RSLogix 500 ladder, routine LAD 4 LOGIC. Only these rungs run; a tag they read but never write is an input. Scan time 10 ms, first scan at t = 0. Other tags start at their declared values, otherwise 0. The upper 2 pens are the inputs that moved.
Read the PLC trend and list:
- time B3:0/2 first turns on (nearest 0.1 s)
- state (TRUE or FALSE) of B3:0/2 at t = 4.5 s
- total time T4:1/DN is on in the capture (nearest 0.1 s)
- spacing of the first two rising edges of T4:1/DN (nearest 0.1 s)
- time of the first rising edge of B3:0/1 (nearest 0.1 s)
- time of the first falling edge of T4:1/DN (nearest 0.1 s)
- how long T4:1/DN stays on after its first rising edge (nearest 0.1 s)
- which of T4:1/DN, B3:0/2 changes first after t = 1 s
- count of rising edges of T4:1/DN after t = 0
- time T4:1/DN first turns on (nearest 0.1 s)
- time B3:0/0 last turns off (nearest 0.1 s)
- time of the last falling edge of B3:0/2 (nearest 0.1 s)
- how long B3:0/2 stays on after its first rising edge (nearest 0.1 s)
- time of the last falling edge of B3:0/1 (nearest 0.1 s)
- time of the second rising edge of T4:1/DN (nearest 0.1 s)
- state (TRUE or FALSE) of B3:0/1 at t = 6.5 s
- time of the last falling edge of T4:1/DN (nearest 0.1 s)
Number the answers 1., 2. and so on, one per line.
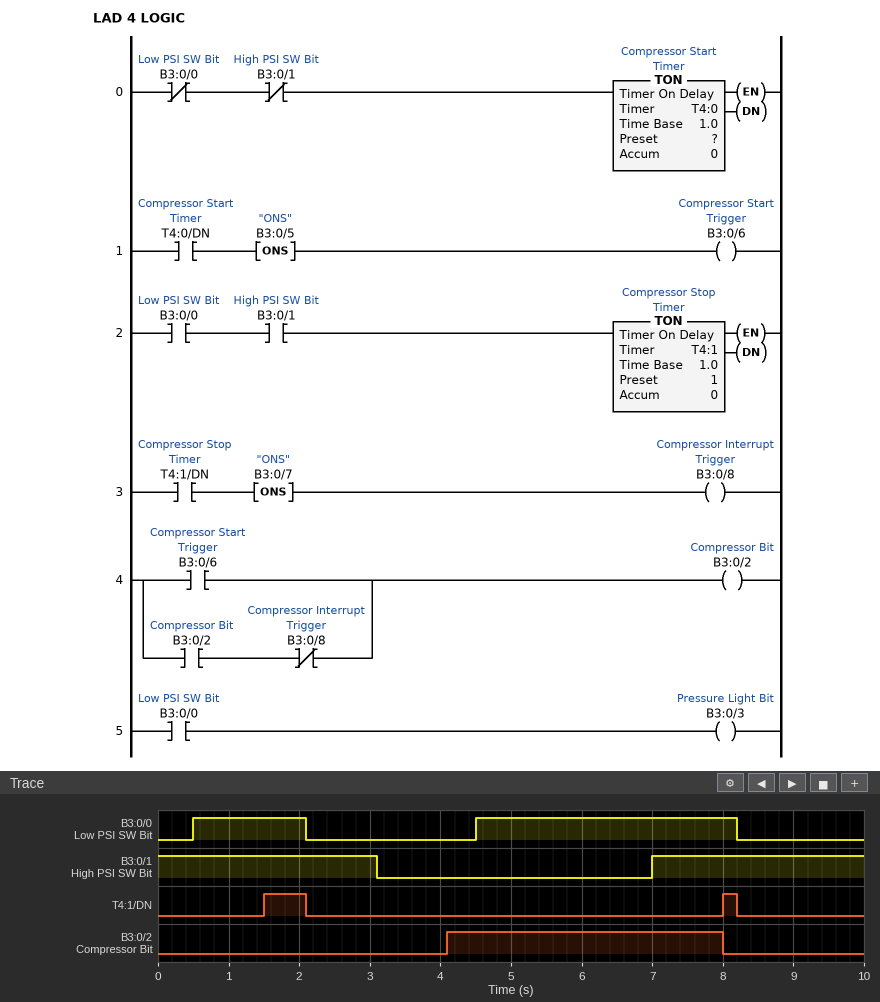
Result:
1. 4.1 s
2. TRUE
3. 0.8 s
4. 6.5 s
5. 7.0 s
6. 2.1 s
7. 0.6 s
8. T4:1/DN
9. 2
10. 1.5 s
11. 8.2 s
12. 8.0 s
13. 3.9 s
14. 3.1 s
15. 8.0 s
16. FALSE
17. 8.2 s
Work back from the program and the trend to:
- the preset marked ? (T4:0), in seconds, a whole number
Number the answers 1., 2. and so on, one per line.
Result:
1. 1 s
